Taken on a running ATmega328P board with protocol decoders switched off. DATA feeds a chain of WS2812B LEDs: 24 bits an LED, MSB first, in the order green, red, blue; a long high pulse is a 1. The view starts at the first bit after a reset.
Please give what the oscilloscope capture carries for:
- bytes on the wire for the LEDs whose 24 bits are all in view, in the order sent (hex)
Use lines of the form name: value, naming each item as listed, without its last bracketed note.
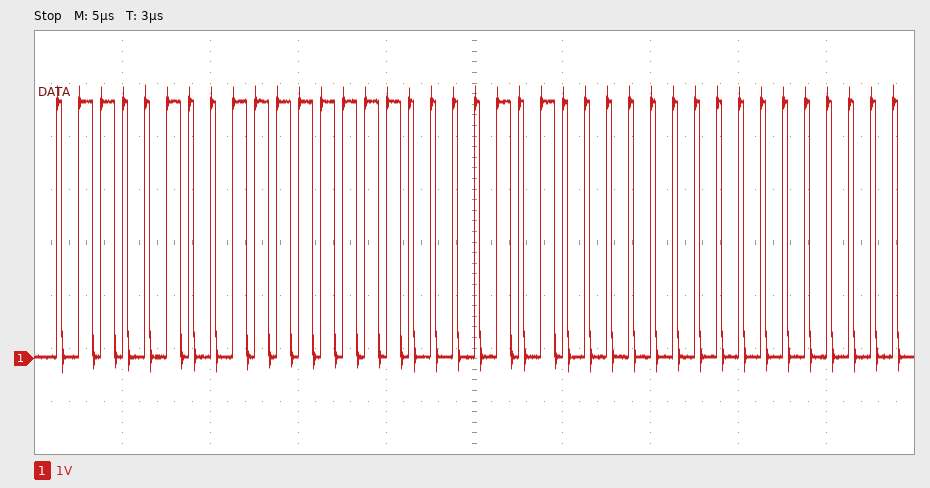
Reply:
bytes on the wire for the LEDs whose 24 bits are all in view, in the order sent: 64 FF 0A
